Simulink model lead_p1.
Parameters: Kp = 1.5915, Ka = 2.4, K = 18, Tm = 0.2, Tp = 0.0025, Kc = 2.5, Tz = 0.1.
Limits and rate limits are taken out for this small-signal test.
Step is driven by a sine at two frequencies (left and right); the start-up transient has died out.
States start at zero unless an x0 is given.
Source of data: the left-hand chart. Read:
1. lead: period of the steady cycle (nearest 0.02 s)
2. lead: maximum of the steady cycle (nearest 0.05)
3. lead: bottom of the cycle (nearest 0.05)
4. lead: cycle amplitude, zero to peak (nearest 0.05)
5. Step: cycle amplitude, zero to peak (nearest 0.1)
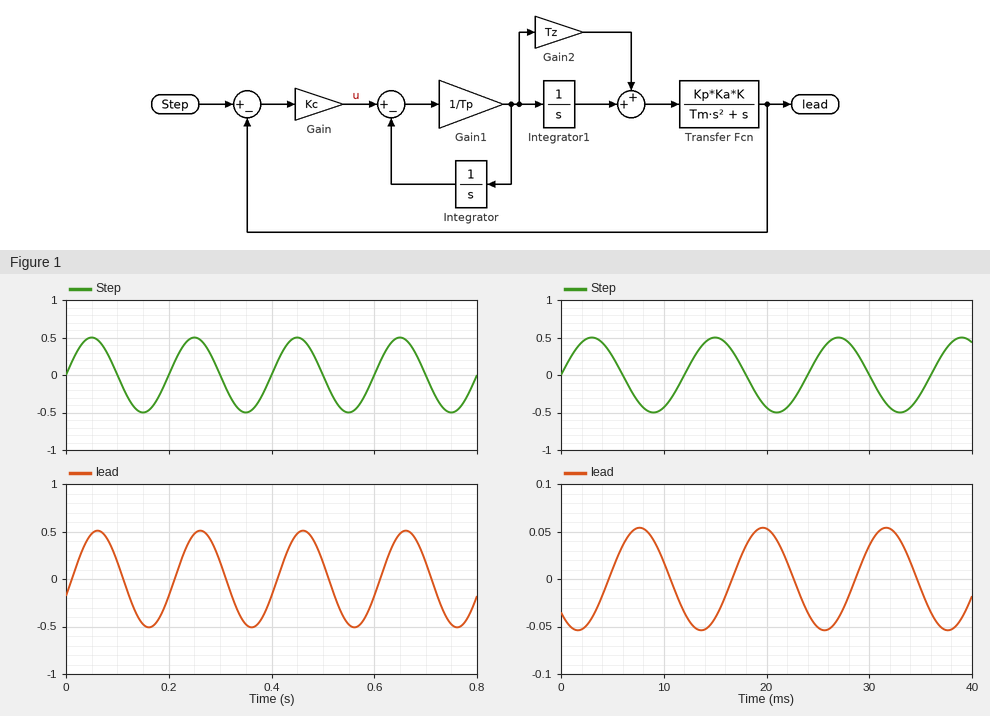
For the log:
0.20 s
0.50
-0.50
0.50
0.5
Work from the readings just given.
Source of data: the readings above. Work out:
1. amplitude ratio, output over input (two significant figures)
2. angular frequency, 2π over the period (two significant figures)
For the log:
1.0
31 rad/s
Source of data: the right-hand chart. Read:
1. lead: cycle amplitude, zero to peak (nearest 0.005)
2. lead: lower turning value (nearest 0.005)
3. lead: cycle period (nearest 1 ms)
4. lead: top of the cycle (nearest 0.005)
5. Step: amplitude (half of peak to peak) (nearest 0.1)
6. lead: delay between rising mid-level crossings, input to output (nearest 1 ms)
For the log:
0.055
-0.055
12 ms
0.055
0.5
5 ms
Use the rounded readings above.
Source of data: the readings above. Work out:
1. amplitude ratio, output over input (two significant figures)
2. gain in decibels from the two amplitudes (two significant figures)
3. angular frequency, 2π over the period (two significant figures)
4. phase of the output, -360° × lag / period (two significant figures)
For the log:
0.11
-19 dB
0.52 rad/ms
-150°
